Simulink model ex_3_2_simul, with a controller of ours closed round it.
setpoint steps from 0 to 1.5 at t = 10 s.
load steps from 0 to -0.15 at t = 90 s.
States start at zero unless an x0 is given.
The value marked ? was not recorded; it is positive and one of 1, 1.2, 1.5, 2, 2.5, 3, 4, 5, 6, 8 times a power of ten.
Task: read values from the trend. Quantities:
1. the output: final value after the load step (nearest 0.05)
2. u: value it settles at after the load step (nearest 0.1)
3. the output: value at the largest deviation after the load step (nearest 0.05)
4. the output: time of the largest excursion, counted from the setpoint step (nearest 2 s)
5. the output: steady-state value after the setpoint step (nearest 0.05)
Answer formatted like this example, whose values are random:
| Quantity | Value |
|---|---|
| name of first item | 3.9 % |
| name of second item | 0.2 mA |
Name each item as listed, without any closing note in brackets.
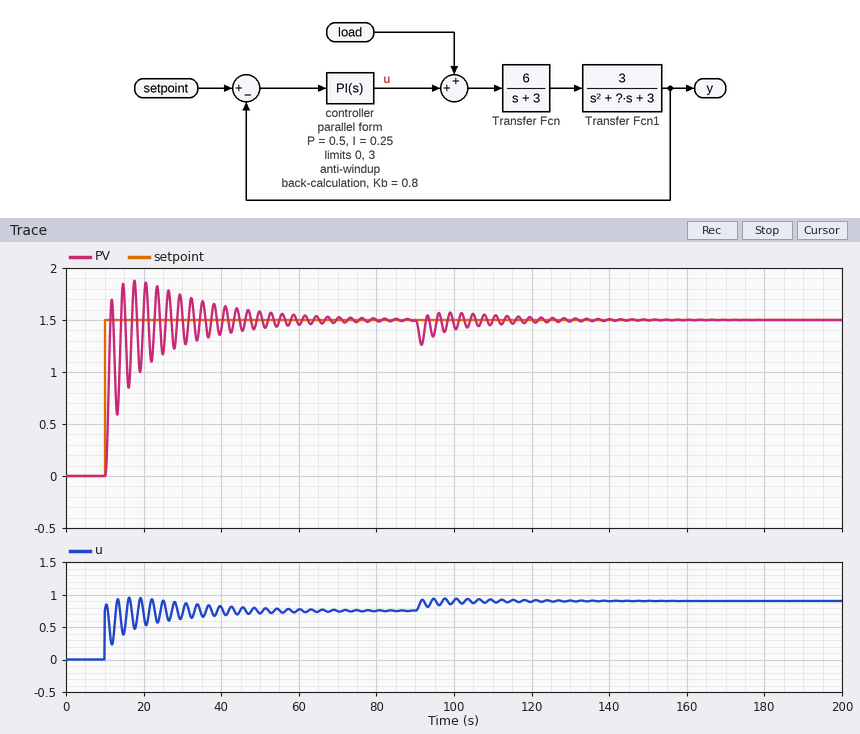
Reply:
| Quantity | Value |
|---|---|
| the output: final value after the load step | 1.50 |
| u: value it settles at after the load step | 0.9 |
| the output: value at the largest deviation after the load step | 1.25 |
| the output: time of the largest excursion, counted from the setpoint step | 8 s |
| the output: steady-state value after the setpoint step | 1.50 |
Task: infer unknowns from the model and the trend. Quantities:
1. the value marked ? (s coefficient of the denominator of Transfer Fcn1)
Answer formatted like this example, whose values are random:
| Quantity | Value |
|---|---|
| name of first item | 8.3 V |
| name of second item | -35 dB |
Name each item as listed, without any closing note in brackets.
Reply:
| Quantity | Value |
|---|---|
| the value marked ? | 1 |
